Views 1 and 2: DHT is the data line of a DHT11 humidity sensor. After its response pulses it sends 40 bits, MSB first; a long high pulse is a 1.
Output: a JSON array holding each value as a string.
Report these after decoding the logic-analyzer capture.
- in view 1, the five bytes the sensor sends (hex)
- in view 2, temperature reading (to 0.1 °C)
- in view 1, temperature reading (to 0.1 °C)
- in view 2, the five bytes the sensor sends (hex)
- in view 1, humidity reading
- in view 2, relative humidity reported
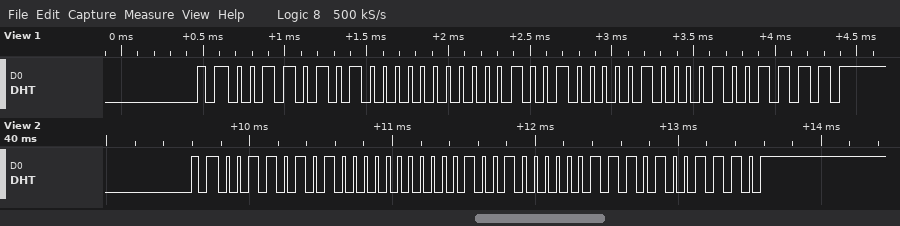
["35 00 12 08 4F", "18.7 °C", "18.8 °C", "35 00 12 07 4E", "53 %", "53 %"]
